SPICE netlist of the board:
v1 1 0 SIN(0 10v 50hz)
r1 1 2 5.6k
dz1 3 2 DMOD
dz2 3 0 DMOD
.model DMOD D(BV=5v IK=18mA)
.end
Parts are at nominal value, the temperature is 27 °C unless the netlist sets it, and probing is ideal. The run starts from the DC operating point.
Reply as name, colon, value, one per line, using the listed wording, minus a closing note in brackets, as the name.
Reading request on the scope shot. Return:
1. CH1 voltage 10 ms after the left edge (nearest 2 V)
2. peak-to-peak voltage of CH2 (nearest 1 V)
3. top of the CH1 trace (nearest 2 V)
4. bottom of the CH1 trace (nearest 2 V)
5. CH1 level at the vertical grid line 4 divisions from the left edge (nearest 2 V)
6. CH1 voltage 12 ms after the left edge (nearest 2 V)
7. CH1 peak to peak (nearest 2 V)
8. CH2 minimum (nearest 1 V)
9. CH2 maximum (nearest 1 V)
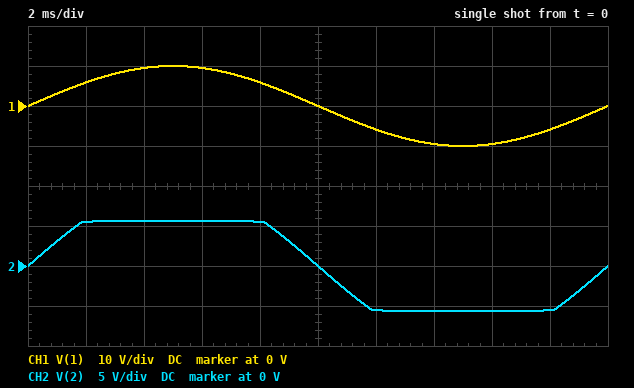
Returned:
CH1 voltage 10 ms after the left edge: 0 V
peak-to-peak voltage of CH2: 11 V
top of the CH1 trace: 10 V
bottom of the CH1 trace: -10 V
CH1 level at the vertical grid line 4 divisions from the left edge: 6 V
CH1 voltage 12 ms after the left edge: -6 V
CH1 peak to peak: 20 V
CH2 minimum: -6 V
CH2 maximum: 6 V
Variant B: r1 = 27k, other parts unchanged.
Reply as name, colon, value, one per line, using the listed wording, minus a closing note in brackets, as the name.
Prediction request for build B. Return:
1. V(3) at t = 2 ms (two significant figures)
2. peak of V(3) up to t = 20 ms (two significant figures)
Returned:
V(3) at t = 2 ms: 550 mV
peak of V(3) up to t = 20 ms: 610 mV
